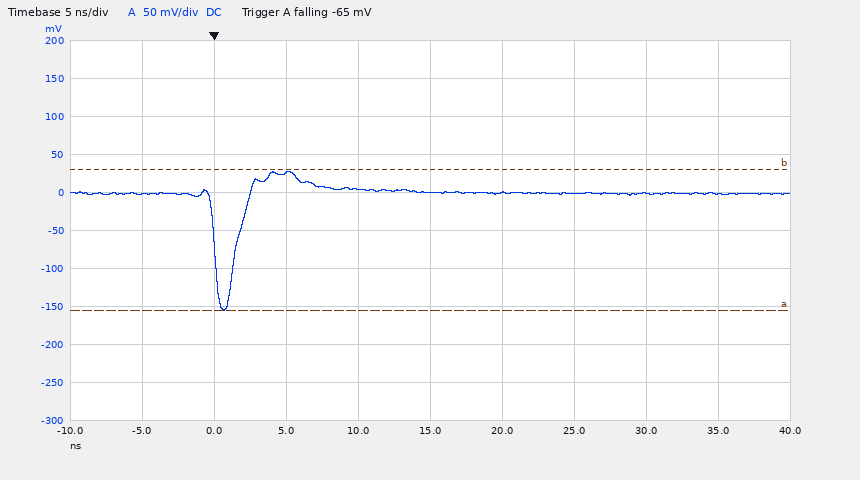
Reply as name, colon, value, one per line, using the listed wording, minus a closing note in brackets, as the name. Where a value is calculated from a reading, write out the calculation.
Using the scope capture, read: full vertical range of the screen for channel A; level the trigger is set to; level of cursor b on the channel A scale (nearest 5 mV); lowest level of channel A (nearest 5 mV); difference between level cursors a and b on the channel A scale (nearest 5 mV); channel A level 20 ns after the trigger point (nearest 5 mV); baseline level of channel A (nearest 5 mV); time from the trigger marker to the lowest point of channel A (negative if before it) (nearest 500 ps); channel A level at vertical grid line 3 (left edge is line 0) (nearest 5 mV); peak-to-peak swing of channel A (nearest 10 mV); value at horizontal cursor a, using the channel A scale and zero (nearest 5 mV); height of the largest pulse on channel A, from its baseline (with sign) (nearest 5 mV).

full vertical range of the screen for channel A: 500 mV
level the trigger is set to: -65 mV
level of cursor b on the channel A scale: 30 mV
lowest level of channel A: -155 mV
difference between level cursors a and b on the channel A scale: 185 mV
channel A level 20 ns after the trigger point: 0 mV
baseline level of channel A: 0 mV
time from the trigger marker to the lowest point of channel A (negative if before it): +500 ps
channel A level at vertical grid line 3 (left edge is line 0): 25 mV
peak-to-peak swing of channel A: 180 mV
value at horizontal cursor a, using the channel A scale and zero: -155 mV
height of the largest pulse on channel A, from its baseline (with sign): -155 mV − (0 mV) = -155 mV
